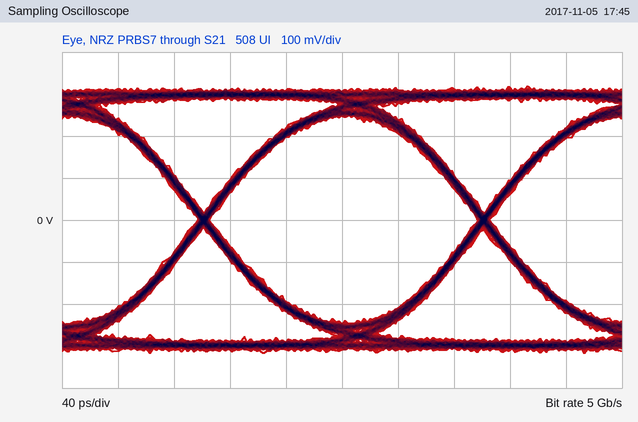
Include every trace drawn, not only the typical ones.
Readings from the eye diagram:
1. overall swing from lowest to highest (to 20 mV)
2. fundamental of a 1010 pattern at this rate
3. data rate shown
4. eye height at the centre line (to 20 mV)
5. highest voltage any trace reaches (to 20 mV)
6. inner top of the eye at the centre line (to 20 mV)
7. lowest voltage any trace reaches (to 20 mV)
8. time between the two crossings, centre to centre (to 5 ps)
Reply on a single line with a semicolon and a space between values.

640 mV; 2.5 GHz; 5 Gb/s; 500 mV; 320 mV; 240 mV; -320 mV; 200 ps
